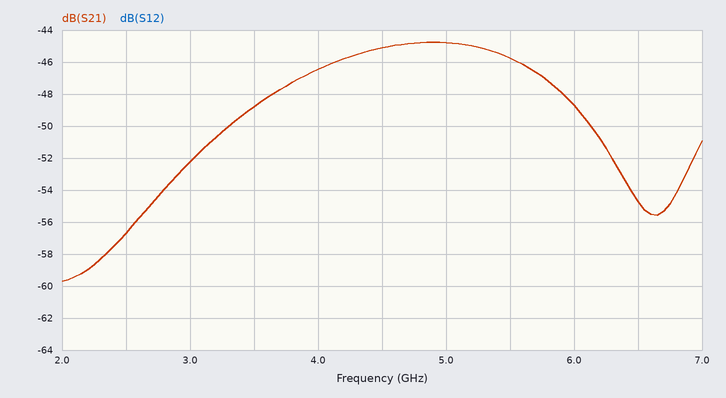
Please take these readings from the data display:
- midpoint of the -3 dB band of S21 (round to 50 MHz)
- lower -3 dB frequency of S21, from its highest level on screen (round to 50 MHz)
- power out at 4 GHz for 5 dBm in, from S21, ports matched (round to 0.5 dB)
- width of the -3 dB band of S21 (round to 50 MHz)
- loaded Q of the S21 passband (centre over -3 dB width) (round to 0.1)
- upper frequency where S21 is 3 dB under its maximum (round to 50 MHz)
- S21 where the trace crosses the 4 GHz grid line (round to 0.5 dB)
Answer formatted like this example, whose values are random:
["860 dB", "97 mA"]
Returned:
["4.80 GHz", "3.70 GHz", "-41.5 dBm", "2.20 GHz", "2.2", "5.90 GHz", "-46.5 dB"]
